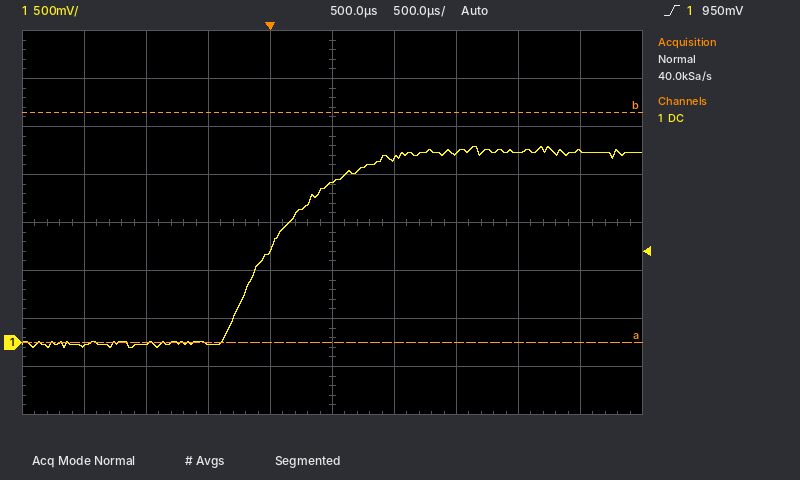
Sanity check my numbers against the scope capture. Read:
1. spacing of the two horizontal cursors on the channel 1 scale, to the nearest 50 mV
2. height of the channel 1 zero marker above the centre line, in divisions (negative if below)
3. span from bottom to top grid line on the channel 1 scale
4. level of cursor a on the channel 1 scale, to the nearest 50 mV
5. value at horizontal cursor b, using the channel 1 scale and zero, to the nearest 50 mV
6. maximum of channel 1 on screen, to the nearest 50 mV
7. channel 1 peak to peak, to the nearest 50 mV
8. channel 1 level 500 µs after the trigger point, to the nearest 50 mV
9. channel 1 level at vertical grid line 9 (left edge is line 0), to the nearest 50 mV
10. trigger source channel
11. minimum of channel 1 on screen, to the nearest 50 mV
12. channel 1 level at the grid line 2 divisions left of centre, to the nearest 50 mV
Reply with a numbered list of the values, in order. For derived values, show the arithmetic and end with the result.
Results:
1. 2.40 V
2. -2.5 div
3. 4 V
4. 0 mV
5. 2.40 V
6. 2.05 V
7. 2.05 V − (-50 mV) = 2.10 V
8. 1.65 V
9. 2.00 V
10. channel 1
11. -50 mV
12. 0 mV
